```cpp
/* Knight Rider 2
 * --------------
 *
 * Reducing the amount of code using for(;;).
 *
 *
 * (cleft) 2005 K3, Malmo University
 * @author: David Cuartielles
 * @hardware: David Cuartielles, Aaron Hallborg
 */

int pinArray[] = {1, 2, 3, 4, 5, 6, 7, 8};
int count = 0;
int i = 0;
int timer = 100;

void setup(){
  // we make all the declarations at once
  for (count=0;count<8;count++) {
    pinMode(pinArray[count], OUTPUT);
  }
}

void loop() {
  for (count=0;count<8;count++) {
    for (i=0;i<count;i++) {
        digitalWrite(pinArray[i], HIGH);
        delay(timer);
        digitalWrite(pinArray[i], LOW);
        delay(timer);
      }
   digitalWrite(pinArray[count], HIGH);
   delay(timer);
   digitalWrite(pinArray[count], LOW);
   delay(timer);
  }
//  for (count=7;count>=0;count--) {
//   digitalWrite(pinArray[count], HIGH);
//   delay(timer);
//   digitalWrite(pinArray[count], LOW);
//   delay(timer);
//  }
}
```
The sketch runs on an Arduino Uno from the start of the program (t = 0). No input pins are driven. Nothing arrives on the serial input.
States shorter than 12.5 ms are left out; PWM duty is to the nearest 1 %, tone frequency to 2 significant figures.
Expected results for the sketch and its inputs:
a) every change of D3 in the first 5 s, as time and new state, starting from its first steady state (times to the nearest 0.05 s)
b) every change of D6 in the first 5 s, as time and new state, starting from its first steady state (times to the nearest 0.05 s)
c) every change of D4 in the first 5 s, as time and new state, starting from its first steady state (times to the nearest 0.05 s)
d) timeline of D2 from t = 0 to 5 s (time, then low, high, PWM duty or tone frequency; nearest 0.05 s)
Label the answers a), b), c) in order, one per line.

a) 0 s low; 1 s high; 1.1 s low; 1.6 s high; 1.7 s low; 2.4 s high; 2.5 s low; 3.4 s high; 3.5 s low; 4.6 s high; 4.7 s low
b) 0 s low; 4 s high; 4.1 s low
c) 0 s low; 1.8 s high; 1.9 s low; 2.6 s high; 2.7 s low; 3.6 s high; 3.7 s low; 4.8 s high; 4.9 s low
d) 0 s low; 0.4 s high; 0.5 s low; 0.8 s high; 0.9 s low; 1.4 s high; 1.5 s low; 2.2 s high; 2.3 s low; 3.2 s high; 3.3 s low; 4.4 s high; 4.5 s low
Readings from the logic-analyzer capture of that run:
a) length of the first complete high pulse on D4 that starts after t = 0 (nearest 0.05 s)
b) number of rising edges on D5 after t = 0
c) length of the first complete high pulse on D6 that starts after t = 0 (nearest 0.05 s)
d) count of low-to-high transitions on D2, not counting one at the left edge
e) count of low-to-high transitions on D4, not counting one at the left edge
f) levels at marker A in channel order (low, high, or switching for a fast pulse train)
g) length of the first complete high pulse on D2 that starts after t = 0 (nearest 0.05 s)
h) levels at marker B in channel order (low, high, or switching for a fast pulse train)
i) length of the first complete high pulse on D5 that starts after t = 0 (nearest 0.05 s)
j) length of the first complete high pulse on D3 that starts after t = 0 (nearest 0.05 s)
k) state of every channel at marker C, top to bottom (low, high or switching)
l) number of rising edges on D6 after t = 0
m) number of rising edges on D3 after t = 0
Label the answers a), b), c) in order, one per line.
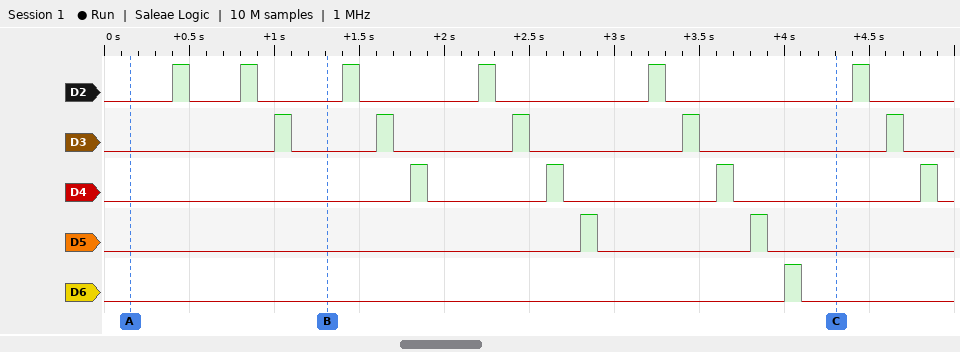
a) 0.10 s
b) 2
c) 0.10 s
d) 6
e) 4
f) D2 low, D3 low, D4 low, D5 low, D6 low
g) 0.10 s
h) D2 low, D3 low, D4 low, D5 low, D6 low
i) 0.10 s
j) 0.10 s
k) D2 low, D3 low, D4 low, D5 low, D6 low
l) 1
m) 5
